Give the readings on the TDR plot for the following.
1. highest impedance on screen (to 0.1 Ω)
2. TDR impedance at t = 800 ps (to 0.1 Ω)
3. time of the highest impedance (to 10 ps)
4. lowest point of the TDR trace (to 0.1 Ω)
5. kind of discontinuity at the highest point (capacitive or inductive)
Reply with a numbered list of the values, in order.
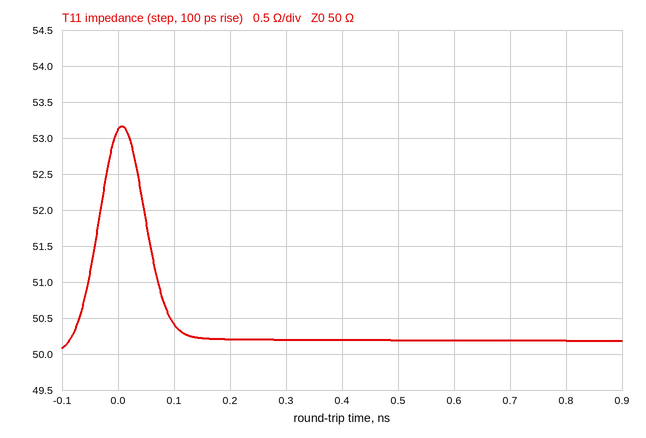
1. 53.2 Ω
2. 50.2 Ω
3. 10 ps
4. 50.1 Ω
5. inductive
